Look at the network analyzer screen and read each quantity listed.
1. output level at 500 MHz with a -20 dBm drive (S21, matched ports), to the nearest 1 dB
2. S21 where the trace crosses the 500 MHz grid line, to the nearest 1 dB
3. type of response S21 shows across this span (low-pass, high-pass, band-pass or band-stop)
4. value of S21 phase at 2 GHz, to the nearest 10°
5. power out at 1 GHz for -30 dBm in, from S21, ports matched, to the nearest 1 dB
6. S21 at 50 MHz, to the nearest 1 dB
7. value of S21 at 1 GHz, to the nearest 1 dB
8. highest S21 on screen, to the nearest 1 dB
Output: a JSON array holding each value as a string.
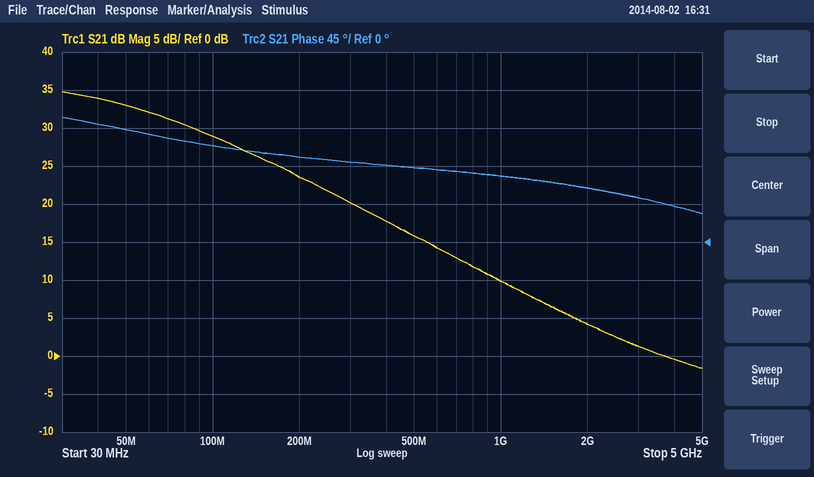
["-4 dBm", "16 dB", "low-pass", "60°", "-20 dBm", "33 dB", "10 dB", "35 dB"]
